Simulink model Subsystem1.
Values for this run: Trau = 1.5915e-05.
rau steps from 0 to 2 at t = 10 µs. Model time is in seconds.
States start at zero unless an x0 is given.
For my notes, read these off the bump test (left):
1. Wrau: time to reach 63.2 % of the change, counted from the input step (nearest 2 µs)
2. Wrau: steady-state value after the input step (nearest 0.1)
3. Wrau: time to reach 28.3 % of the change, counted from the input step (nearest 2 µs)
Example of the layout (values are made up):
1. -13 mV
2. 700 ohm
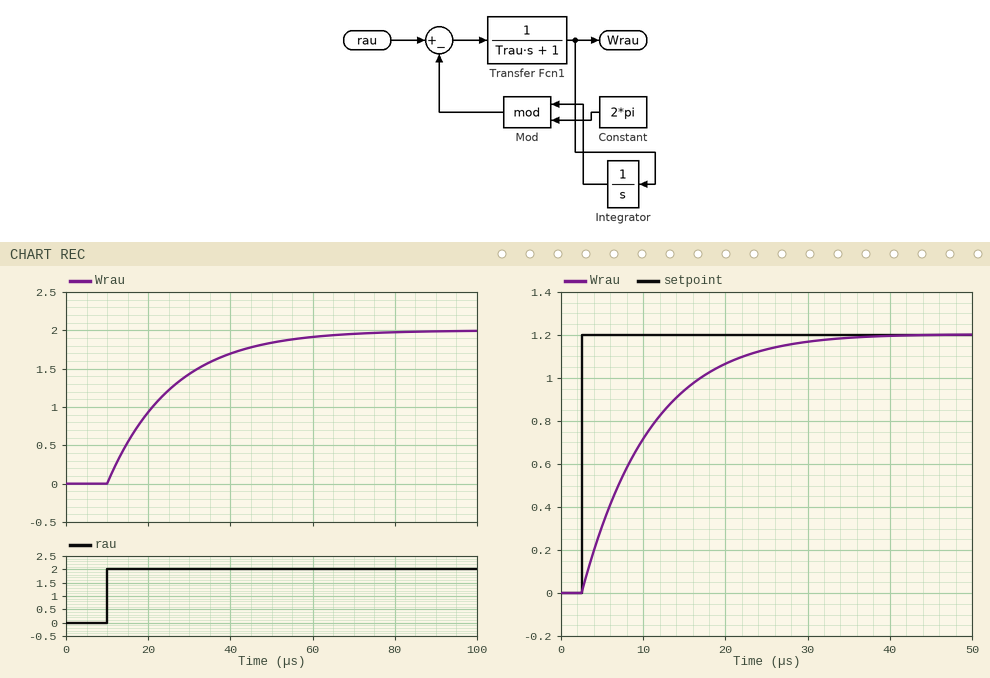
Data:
1. 16 µs
2. 2.0
3. 6 µs
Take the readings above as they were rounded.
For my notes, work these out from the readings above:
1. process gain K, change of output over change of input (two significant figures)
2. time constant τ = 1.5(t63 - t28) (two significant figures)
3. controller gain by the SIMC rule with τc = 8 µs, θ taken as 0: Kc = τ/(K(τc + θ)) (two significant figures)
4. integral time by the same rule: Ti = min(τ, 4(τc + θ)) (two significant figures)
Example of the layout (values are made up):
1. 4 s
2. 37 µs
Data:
1. 1.0
2. 15 µs
3. 1.9
4. 15 µs
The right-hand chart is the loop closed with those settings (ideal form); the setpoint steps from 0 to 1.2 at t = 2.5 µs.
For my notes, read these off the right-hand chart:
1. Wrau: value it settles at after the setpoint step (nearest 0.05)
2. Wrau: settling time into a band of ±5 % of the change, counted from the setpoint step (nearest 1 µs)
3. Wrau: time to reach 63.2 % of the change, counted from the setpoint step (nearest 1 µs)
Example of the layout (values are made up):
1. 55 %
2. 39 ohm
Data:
1. 1.20
2. 23 µs
3. 8 µs
